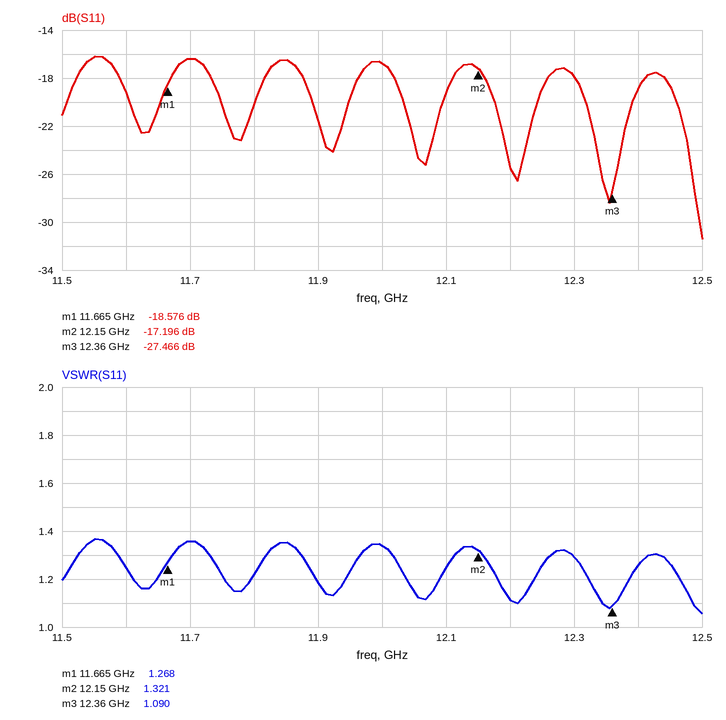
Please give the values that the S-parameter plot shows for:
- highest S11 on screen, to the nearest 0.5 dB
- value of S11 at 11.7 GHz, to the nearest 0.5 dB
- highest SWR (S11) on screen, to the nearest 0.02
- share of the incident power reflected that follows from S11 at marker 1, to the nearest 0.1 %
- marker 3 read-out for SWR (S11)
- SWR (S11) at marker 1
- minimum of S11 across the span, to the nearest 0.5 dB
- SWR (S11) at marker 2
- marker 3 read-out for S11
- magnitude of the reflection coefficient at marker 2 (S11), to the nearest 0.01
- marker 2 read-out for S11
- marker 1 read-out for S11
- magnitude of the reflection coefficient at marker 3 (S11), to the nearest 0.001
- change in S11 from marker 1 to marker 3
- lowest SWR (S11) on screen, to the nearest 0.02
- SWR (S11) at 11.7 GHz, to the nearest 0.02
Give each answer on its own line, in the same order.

-16.0 dB
-16.5 dB
1.36
1.4 %
1.090
1.268
-31.5 dB
1.321
-27.466 dB
0.14
-17.196 dB
-18.576 dB
0.042
-8.890 dB
1.06
1.36
